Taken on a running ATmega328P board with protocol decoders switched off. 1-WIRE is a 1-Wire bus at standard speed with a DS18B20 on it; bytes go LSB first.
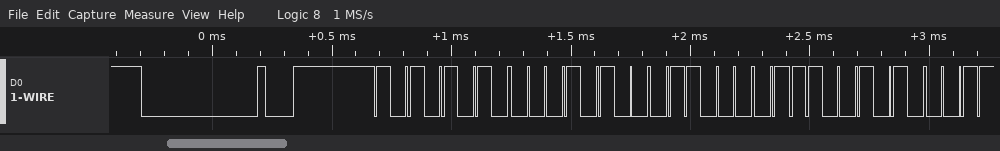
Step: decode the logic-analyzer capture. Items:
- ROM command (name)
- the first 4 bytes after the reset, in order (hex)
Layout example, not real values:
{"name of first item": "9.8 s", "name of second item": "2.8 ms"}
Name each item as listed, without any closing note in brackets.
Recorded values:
{"ROM command": "Match ROM", "the first 4 bytes after the reset, in order": "55 28 86 53"}
